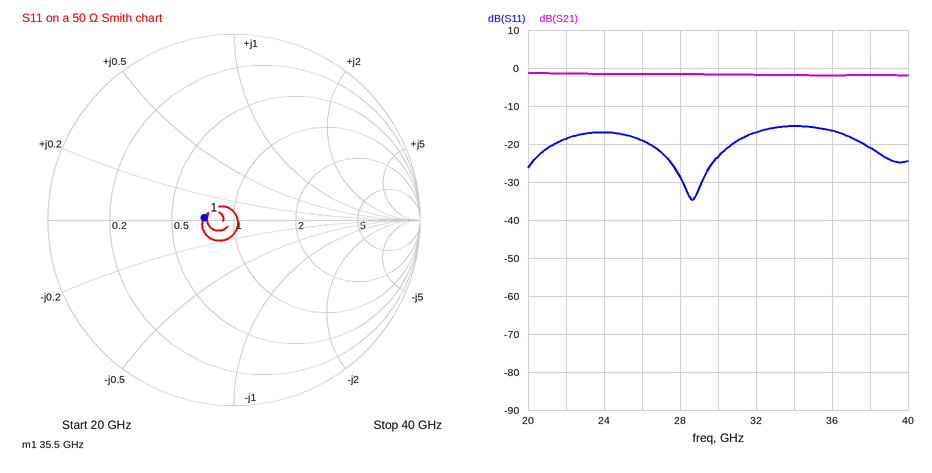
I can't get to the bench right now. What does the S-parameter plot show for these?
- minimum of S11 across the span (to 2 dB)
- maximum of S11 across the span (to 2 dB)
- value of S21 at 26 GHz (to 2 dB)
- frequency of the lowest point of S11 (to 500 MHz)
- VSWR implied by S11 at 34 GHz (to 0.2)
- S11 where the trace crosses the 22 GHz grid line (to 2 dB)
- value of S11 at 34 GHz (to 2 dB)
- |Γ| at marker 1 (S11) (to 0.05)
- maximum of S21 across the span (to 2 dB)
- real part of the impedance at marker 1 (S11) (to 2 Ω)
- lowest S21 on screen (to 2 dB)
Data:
-34 dB
-16 dB
-2 dB
28.5 GHz
1.4
-18 dB
-16 dB
0.15
-2 dB
36 Ω
-2 dB
